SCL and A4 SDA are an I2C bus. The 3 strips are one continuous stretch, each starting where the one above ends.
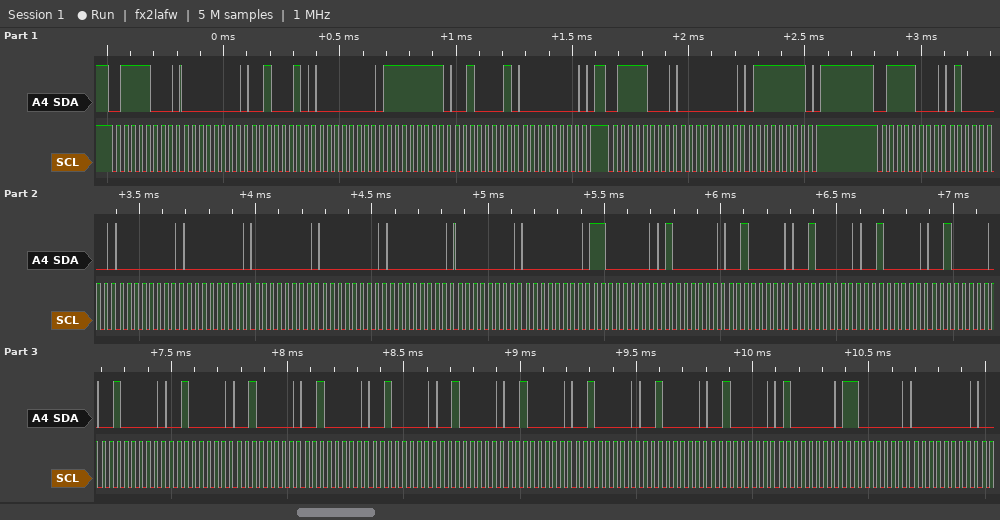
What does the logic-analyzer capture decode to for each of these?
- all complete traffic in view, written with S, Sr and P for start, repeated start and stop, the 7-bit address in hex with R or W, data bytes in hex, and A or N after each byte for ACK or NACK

S 3CW A 00 A 22 A 00 A FF A 21 A 00 A P S 3CW A 00 A 7F A P S 3CW A 40 A 00 A 00 A 00 A 00 A 00 A 00 A 00 A C0 A 40 A 20 A 20 A 20 A 20 A 20 A 20 A 20 A 20 A 20 A 20 A 20 A 20 A 20 A 20 A 40 A C0 A 00 A
